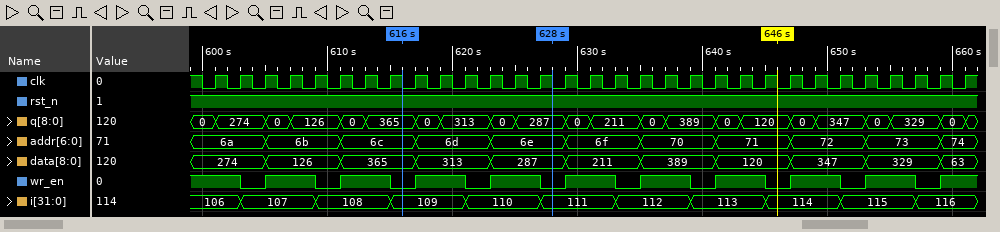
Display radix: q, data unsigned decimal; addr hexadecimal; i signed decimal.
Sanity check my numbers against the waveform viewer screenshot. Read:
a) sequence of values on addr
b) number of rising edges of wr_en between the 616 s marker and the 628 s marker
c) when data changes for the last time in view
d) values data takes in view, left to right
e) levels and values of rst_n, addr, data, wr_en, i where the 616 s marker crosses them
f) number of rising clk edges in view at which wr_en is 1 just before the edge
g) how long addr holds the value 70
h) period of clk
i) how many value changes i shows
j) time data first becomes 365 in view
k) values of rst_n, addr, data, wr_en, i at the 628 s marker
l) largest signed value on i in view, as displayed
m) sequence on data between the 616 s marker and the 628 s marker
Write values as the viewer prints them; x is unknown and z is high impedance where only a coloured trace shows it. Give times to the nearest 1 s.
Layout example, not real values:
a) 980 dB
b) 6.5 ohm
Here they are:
a) 6a, 6b, 6c, 6d, 6e, 6f, 70, 71, 72, 73, 74
b) 2
c) 659 s
d) 274, 126, 365, 313, 287, 211, 389, 120, 347, 329, 63
e) rst_n=1, addr=6c, data=365, wr_en=0, i=109
f) 21
g) 6 s
h) 2 s
i) 10
j) 611 s
k) rst_n=1, addr=6e, data=287, wr_en=0, i=111
l) 116
m) 365, 313, 287
